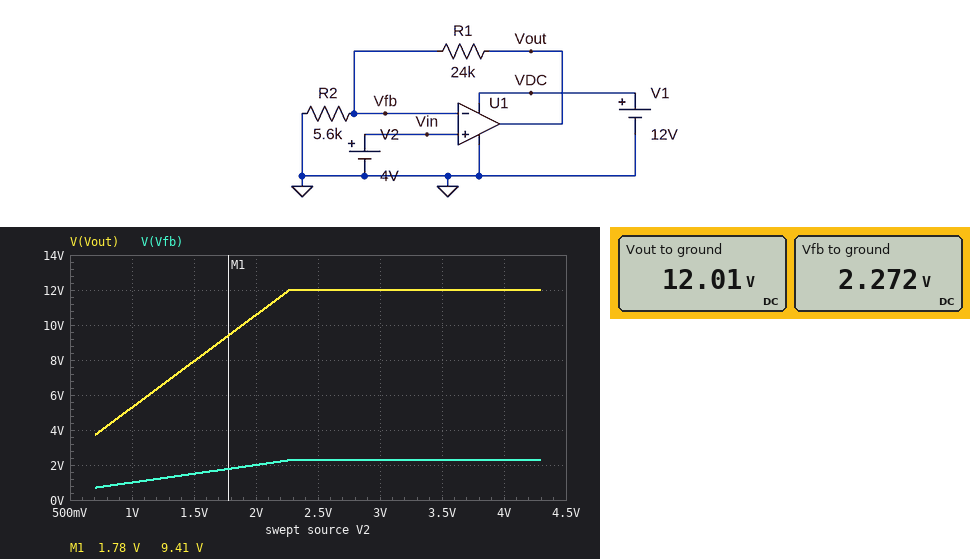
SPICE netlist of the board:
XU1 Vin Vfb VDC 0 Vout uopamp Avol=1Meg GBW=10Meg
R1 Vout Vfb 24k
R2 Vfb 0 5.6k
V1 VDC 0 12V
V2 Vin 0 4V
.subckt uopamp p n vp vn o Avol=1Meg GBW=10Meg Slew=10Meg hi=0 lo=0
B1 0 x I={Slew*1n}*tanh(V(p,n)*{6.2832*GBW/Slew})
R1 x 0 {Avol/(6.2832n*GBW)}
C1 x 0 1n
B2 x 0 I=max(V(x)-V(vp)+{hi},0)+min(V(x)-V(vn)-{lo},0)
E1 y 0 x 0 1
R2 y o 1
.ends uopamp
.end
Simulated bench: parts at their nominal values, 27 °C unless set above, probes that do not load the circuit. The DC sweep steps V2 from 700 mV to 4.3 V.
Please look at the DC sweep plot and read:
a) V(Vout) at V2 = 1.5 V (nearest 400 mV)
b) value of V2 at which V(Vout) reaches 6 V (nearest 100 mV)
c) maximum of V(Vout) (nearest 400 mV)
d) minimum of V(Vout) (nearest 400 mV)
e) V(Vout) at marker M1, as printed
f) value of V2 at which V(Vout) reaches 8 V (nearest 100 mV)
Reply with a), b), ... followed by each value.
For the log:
a) 8.0 V
b) 1.1 V
c) 12.0 V
d) 3.6 V
e) 9.41 V
f) 1.5 V
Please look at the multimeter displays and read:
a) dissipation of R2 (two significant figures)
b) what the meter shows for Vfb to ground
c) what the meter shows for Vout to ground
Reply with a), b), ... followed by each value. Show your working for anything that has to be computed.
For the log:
a) (2.272 V)^2 / 5.6 kΩ = 920 µW
b) 2.272 V
c) 12.01 V
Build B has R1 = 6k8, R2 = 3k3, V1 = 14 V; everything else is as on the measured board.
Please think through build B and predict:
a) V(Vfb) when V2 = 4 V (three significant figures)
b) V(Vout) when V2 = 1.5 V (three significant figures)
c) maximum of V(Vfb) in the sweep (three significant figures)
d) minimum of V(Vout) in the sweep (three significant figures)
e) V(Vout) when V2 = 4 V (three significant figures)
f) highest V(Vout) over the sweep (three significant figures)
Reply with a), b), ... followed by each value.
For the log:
a) 4.00 V
b) 4.59 V
c) 4.30 V
d) 2.14 V
e) 12.2 V
f) 13.2 V
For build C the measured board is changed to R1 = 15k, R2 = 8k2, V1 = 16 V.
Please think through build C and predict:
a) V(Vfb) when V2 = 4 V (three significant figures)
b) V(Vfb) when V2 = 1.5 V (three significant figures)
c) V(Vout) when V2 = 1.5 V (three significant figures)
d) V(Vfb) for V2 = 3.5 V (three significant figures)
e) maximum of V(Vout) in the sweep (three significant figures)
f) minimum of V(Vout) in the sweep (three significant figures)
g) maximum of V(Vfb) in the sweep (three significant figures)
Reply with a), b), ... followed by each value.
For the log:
a) 4.00 V
b) 1.50 V
c) 4.24 V
d) 3.50 V
e) 12.2 V
f) 1.98 V
g) 4.30 V
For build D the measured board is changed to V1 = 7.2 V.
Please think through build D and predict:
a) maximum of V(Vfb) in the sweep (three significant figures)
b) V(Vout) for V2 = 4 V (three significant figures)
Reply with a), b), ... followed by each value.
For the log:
a) 1.36 V
b) 7.21 V
